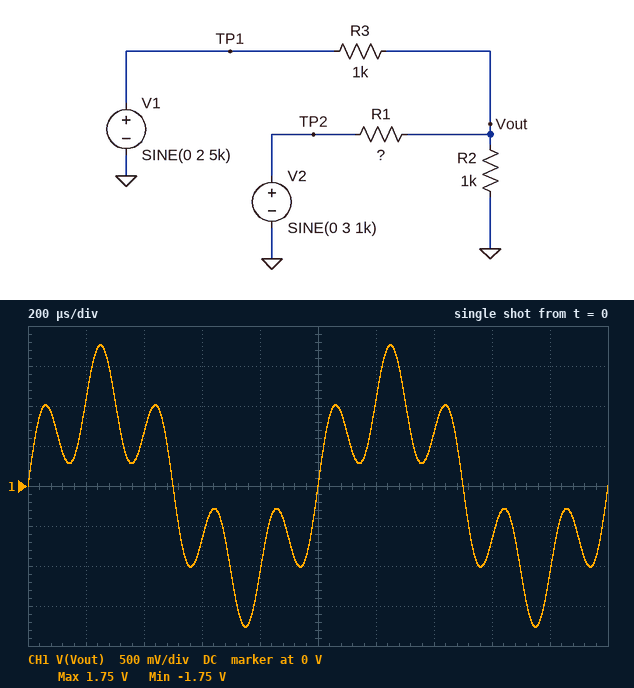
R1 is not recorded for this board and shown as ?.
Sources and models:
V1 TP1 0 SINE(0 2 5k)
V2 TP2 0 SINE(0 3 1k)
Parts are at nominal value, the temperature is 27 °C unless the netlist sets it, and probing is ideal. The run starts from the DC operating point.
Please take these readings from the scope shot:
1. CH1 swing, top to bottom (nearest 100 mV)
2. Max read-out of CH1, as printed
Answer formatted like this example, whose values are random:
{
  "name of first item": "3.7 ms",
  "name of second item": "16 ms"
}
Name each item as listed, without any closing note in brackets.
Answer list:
{
  "CH1 swing, top to bottom": "3.5 V",
  "Max read-out of CH1, as printed": "1.75 V"
}
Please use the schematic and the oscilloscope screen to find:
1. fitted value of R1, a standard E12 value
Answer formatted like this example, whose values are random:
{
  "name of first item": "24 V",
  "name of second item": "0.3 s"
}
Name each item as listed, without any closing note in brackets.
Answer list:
{
  "fitted value of R1, a standard E12 value": "820 Ω"
}
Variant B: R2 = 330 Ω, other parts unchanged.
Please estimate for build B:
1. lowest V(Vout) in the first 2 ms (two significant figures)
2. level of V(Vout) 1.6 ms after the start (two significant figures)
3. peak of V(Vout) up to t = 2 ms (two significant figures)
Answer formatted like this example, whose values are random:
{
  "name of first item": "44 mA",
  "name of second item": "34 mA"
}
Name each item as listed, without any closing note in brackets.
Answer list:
{
  "lowest V(Vout) in the first 2 ms": "-1.1 V",
  "level of V(Vout) 1.6 ms after the start": "-410 mV",
  "peak of V(Vout) up to t = 2 ms": "1.1 V"
}
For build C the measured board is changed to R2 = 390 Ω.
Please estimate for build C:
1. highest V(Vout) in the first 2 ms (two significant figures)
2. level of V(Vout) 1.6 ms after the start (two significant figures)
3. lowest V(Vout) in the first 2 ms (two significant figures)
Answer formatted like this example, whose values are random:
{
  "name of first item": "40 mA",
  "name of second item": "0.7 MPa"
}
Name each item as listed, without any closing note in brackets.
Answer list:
{
  "highest V(Vout) in the first 2 ms": "1.2 V",
  "level of V(Vout) 1.6 ms after the start": "-450 mV",
  "lowest V(Vout) in the first 2 ms": "-1.2 V"
}
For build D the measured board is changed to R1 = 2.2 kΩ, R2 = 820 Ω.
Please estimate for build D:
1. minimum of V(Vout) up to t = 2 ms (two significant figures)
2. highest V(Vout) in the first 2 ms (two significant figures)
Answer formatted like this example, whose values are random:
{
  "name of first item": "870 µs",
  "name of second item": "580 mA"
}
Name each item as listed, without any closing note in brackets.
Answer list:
{
  "minimum of V(Vout) up to t = 2 ms": "-1.3 V",
  "highest V(Vout) in the first 2 ms": "1.3 V"
}
